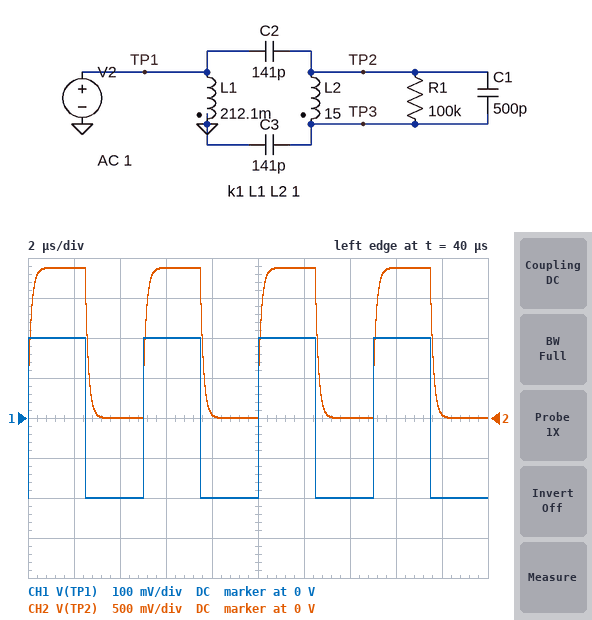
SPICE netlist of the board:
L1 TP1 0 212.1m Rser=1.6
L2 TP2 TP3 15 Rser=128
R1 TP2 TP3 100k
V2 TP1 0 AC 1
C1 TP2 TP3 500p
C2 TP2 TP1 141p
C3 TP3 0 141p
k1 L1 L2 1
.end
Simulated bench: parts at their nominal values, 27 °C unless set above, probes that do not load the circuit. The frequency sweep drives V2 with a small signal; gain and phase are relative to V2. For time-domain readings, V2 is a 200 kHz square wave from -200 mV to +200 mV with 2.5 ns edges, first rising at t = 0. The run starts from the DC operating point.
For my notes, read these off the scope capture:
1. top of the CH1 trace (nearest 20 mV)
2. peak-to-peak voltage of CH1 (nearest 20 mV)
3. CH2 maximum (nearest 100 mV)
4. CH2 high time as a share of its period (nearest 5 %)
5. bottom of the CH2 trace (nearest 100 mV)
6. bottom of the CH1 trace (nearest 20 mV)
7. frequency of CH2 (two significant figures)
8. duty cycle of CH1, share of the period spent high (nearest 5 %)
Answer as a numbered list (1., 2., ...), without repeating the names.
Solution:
1. 200 mV
2. 400 mV
3. 1.9 V
4. 50 %
5. 0 V
6. -200 mV
7. 200 kHz
8. 50 %
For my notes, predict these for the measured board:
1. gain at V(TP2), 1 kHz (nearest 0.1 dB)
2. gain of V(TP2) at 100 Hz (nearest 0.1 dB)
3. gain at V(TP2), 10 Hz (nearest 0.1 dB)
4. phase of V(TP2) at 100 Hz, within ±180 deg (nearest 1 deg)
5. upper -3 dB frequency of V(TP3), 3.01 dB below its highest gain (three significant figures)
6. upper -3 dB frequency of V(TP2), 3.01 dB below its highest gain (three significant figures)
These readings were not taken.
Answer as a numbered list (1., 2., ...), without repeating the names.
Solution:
1. 13.4 dB
2. 13.4 dB
3. 13.4 dB
4. 1 deg
5. 1.18 MHz
6. 1.18 MHz
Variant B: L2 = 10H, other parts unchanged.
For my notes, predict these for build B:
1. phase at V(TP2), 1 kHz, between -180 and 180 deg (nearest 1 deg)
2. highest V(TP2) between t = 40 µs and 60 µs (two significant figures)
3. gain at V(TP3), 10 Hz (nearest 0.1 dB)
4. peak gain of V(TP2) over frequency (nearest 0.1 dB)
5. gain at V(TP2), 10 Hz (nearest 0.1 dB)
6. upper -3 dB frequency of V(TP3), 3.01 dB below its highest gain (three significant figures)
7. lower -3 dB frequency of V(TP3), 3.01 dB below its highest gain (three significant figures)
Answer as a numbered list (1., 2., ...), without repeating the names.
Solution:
1. 0 deg
2. 1.6 V
3. 9.3 dB
4. 11.9 dB
5. 11.8 dB
6. 1.41 MHz
7. 1.16 Hz
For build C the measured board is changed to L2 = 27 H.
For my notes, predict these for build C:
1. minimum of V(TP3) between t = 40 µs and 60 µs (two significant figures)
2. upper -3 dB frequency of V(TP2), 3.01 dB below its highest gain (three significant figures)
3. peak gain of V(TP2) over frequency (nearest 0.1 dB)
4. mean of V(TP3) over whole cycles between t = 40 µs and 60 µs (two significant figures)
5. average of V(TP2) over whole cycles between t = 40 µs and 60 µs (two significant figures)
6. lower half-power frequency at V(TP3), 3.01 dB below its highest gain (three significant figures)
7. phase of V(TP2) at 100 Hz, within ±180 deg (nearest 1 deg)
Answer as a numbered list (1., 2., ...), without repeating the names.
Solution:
1. -2.2 V
2. 851 kHz
3. 15.7 dB
4. -1.0 V
5. 1.2 V
6. 1.19 Hz
7. 1 deg
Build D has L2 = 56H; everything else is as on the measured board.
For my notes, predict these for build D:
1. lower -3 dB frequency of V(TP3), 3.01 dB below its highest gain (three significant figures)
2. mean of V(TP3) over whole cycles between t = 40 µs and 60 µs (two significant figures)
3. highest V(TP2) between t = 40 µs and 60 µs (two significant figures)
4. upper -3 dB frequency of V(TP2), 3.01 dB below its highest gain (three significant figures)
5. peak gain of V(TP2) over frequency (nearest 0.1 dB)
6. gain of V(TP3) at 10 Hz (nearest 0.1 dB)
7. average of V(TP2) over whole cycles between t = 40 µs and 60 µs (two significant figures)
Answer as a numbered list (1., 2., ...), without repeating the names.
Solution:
1. 1.19 Hz
2. -1.5 V
3. 3.4 V
4. 512 kHz
5. 18.7 dB
6. 17.5 dB
7. 1.7 V
